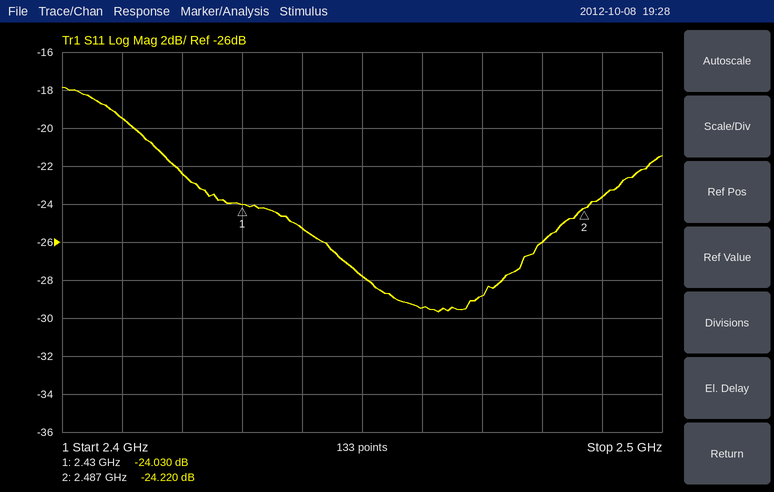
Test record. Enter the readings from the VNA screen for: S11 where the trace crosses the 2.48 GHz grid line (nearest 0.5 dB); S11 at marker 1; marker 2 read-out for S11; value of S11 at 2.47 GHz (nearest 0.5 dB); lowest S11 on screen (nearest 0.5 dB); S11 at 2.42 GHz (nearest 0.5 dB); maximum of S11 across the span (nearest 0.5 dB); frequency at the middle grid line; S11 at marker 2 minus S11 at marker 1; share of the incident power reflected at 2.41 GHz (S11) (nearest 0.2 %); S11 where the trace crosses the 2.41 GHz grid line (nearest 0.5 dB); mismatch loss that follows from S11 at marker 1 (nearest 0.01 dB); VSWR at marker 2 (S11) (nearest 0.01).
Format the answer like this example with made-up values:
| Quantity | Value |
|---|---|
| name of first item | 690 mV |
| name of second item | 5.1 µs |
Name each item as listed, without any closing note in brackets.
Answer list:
| Quantity | Value |
|---|---|
| S11 where the trace crosses the 2.48 GHz grid line | -26.0 dB |
| S11 at marker 1 | -24.030 dB |
| marker 2 read-out for S11 | -24.220 dB |
| value of S11 at 2.47 GHz | -29.0 dB |
| lowest S11 on screen | -29.5 dB |
| S11 at 2.42 GHz | -22.5 dB |
| maximum of S11 across the span | -18.0 dB |
| frequency at the middle grid line | 2.45 GHz |
| S11 at marker 2 minus S11 at marker 1 | -0.190 dB |
| share of the incident power reflected at 2.41 GHz (S11) | 1.2 % |
| S11 where the trace crosses the 2.41 GHz grid line | -19.5 dB |
| mismatch loss that follows from S11 at marker 1 | 0.02 dB |
| VSWR at marker 2 (S11) | 1.13 |
